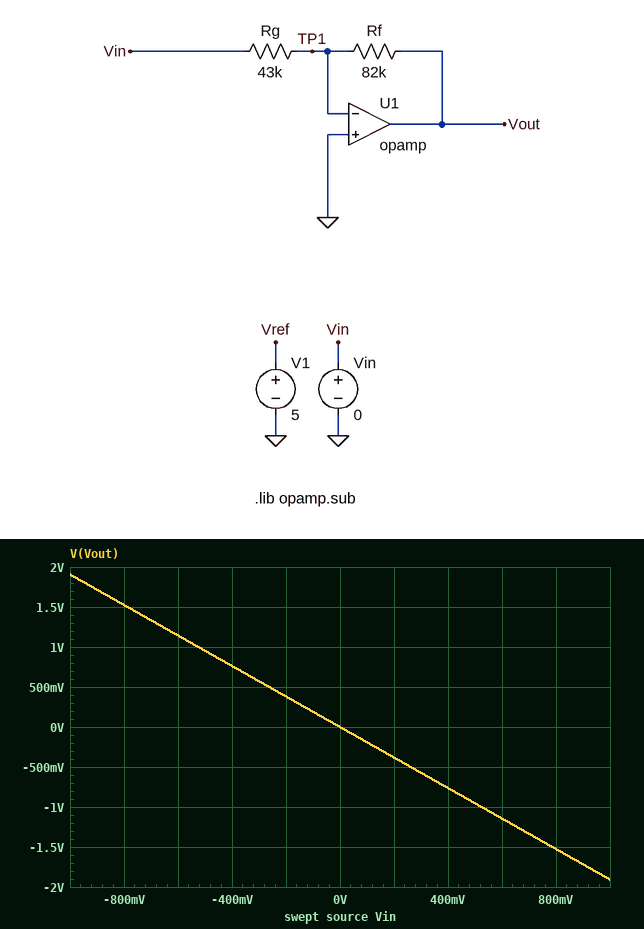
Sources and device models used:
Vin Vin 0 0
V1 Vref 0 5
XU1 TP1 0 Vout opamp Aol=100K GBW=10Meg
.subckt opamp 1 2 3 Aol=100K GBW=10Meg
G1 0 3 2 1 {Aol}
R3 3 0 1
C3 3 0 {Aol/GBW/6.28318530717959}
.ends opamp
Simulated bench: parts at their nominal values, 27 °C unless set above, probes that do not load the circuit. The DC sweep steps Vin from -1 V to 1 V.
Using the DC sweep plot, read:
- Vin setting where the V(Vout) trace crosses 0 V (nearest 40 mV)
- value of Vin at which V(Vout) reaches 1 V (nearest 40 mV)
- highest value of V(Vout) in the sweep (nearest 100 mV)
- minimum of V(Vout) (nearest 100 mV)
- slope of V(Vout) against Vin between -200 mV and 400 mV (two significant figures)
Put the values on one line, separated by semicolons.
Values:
0 V; -520 mV; 1.9 V; -1.9 V; -1.9 V/V
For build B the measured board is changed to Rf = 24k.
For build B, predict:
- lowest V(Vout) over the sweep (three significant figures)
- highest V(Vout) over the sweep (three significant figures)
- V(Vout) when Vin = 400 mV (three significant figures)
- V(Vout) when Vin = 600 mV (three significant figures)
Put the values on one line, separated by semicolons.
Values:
-558 mV; 558 mV; -223 mV; -335 mV
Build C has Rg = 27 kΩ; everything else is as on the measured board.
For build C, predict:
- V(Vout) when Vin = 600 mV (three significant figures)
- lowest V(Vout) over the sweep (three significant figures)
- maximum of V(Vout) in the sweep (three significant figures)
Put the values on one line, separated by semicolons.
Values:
-1.82 V; -3.04 V; 3.04 V
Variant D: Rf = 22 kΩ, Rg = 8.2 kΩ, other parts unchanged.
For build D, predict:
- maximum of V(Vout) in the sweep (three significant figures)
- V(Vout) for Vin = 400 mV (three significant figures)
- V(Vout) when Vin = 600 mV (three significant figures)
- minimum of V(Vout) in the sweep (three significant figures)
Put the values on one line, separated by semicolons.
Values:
2.68 V; -1.07 V; -1.61 V; -2.68 V
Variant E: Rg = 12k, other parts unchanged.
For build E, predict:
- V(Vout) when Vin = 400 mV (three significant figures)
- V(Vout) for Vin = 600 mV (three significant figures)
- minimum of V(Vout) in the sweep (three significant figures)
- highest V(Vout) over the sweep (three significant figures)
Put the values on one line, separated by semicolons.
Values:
-2.73 V; -4.10 V; -6.83 V; 6.83 V
